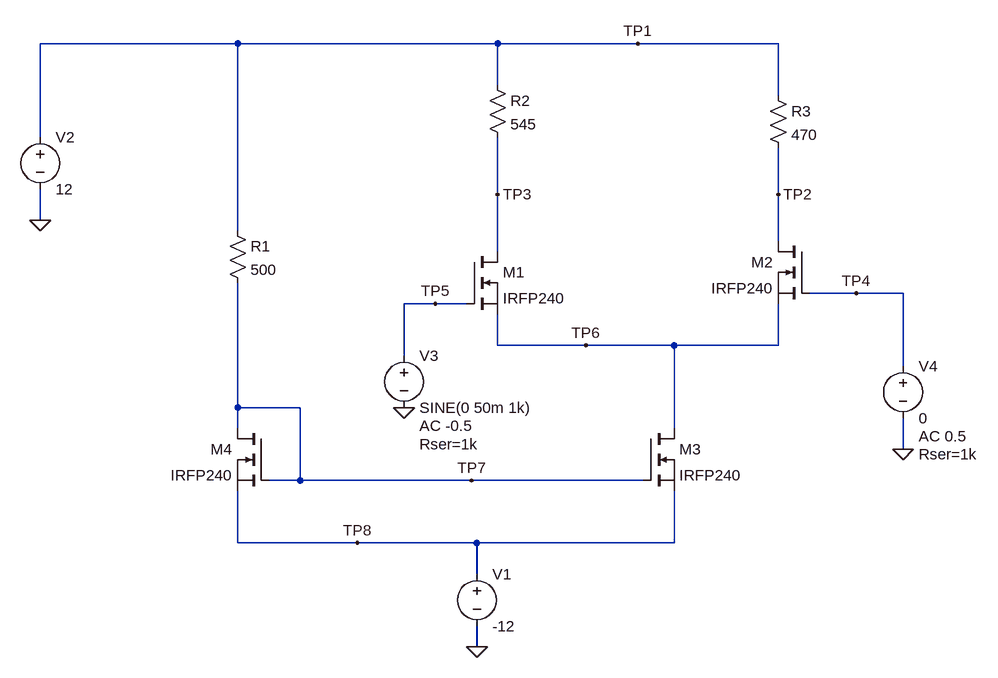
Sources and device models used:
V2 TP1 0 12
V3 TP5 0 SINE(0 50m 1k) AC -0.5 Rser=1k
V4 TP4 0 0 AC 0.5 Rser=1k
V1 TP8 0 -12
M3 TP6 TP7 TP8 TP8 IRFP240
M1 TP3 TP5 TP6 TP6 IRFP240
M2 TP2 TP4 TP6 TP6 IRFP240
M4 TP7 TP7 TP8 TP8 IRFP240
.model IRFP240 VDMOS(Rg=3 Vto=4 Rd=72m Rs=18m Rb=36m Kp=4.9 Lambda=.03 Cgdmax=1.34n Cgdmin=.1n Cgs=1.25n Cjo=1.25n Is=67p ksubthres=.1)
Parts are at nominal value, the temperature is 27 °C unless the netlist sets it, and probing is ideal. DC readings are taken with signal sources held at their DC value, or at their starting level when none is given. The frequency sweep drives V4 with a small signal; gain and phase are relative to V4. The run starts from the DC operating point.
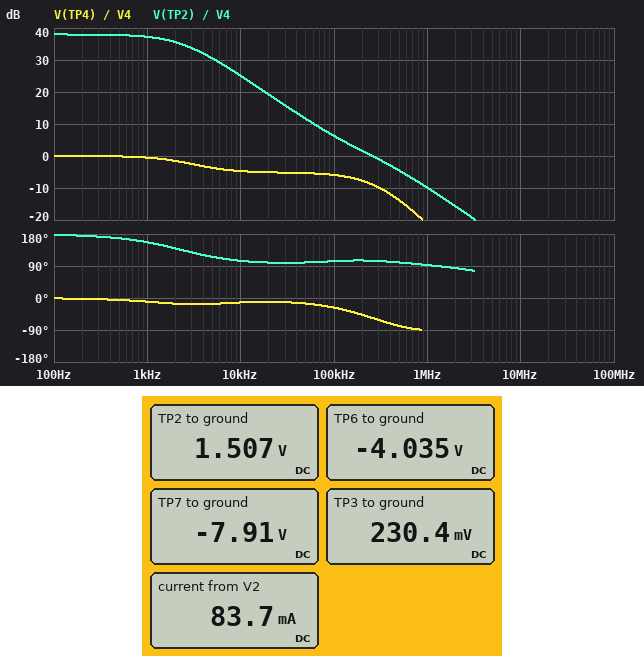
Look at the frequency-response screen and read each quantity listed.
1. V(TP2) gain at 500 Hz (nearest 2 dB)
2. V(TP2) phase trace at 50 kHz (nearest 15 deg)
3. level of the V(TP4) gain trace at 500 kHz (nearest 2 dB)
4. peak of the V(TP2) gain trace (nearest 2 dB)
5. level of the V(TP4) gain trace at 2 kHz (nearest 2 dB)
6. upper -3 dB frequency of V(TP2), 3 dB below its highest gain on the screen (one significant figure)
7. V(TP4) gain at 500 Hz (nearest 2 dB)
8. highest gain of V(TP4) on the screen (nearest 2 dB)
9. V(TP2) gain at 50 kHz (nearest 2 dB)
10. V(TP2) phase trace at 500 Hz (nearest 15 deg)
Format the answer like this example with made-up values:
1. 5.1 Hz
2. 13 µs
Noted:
1. 38 dB
2. 105 deg
3. -14 dB
4. 38 dB
5. -2 dB
6. 2 kHz
7. 0 dB
8. 0 dB
9. 12 dB
10. 165 deg
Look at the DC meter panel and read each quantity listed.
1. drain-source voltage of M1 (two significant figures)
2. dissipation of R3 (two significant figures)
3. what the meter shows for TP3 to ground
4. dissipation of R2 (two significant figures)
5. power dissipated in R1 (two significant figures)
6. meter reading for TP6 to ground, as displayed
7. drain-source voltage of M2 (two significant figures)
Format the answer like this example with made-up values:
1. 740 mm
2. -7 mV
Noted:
1. 4.3 V
2. 230 mW
3. 230.4 mV
4. 250 mW
5. 790 mW
6. -4.035 V
7. 5.5 V
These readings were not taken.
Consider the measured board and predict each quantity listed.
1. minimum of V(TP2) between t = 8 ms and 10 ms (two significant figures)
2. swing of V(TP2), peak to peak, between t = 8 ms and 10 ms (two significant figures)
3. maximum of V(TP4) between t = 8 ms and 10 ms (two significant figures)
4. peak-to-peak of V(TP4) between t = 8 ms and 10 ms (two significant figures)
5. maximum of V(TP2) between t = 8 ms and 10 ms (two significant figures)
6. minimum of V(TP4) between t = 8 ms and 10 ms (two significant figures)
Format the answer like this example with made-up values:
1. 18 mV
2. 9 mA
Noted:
1. -860 mV
2. 4.6 V
3. 11 mV
4. 21 mV
5. 3.8 V
6. -10 mV
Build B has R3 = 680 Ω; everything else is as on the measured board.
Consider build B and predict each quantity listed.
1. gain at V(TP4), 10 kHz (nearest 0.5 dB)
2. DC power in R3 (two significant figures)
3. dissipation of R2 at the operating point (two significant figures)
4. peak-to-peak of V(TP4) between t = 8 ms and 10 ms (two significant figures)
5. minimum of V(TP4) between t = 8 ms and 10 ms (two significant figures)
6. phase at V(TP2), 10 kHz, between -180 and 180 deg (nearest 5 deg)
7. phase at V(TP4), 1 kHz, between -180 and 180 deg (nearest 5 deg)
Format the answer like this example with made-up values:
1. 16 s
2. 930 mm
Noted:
1. -18.0 dB
2. 310 mW
3. 280 mW
4. 41 mV
5. -23 mV
6. 95 deg
7. -40 deg
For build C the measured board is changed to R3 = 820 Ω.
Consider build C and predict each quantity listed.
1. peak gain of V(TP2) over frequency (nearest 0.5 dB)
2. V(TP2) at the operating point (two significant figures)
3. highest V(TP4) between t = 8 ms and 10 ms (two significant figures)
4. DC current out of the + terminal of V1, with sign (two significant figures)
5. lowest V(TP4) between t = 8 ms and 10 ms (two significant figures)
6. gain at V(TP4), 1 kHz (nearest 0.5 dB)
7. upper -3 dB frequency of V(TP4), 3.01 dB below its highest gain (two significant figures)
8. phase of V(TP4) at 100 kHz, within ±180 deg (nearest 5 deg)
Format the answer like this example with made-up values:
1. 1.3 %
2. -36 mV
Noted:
1. 6.0 dB
2. -4.0 V
3. 13 mV
4. -84 mA
5. -22 mV
6. 0 dB
7. 26 kHz
8. -55 deg
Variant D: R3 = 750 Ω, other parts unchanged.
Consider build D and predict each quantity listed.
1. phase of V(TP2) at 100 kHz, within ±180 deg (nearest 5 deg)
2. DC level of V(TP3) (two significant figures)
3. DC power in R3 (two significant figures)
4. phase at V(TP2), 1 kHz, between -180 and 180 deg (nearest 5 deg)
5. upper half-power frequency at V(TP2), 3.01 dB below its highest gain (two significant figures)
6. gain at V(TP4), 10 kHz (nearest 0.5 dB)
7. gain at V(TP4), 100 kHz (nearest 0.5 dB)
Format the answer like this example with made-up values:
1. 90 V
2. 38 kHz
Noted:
1. 85 deg
2. -510 mV
3. 330 mW
4. 135 deg
5. 960 Hz
6. -19.0 dB
7. -21.5 dB
